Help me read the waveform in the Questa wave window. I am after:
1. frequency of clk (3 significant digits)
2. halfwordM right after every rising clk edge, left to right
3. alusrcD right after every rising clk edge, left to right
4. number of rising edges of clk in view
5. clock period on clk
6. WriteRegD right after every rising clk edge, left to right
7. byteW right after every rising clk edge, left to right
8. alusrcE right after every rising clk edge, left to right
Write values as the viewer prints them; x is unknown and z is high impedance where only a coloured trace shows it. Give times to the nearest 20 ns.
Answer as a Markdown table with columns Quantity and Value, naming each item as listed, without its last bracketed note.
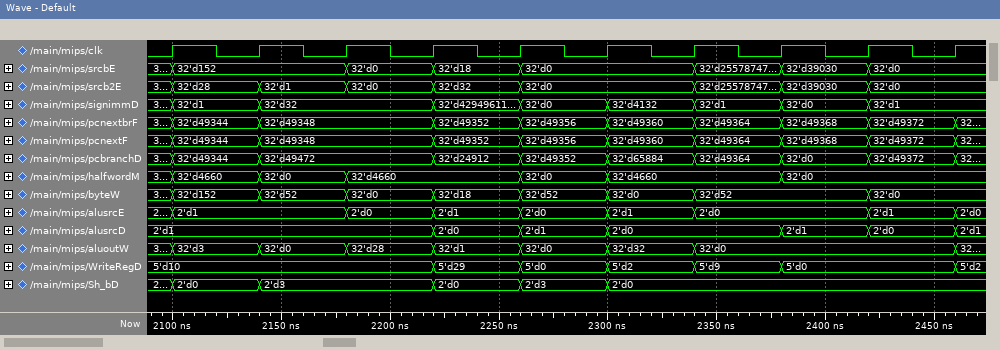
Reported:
| Quantity | Value |
|---|---|
| frequency of clk | 25.0 MHz |
| halfwordM right after every rising clk edge, left to right | 32'd4660, 32'd0, 32'd4660, 32'd4660, 32'd0, 32'd4660, 32'd4660, 32'd0, 32'd0, 32'd0 |
| alusrcD right after every rising clk edge, left to right | 2'd1, 2'd1, 2'd1, 2'd0, 2'd1, 2'd0, 2'd0, 2'd1, 2'd0, 2'd1 |
| number of rising edges of clk in view | 10 |
| clock period on clk | 40 ns |
| WriteRegD right after every rising clk edge, left to right | 5'd10, 5'd10, 5'd10, 5'd29, 5'd0, 5'd2, 5'd9, 5'd0, 5'd0, 5'd2 |
| byteW right after every rising clk edge, left to right | 32'd152, 32'd52, 32'd0, 32'd18, 32'd52, 32'd0, 32'd52, 32'd52, 32'd0, 32'd0 |
| alusrcE right after every rising clk edge, left to right | 2'd1, 2'd1, 2'd0, 2'd1, 2'd0, 2'd1, 2'd0, 2'd0, 2'd1, 2'd0 |
